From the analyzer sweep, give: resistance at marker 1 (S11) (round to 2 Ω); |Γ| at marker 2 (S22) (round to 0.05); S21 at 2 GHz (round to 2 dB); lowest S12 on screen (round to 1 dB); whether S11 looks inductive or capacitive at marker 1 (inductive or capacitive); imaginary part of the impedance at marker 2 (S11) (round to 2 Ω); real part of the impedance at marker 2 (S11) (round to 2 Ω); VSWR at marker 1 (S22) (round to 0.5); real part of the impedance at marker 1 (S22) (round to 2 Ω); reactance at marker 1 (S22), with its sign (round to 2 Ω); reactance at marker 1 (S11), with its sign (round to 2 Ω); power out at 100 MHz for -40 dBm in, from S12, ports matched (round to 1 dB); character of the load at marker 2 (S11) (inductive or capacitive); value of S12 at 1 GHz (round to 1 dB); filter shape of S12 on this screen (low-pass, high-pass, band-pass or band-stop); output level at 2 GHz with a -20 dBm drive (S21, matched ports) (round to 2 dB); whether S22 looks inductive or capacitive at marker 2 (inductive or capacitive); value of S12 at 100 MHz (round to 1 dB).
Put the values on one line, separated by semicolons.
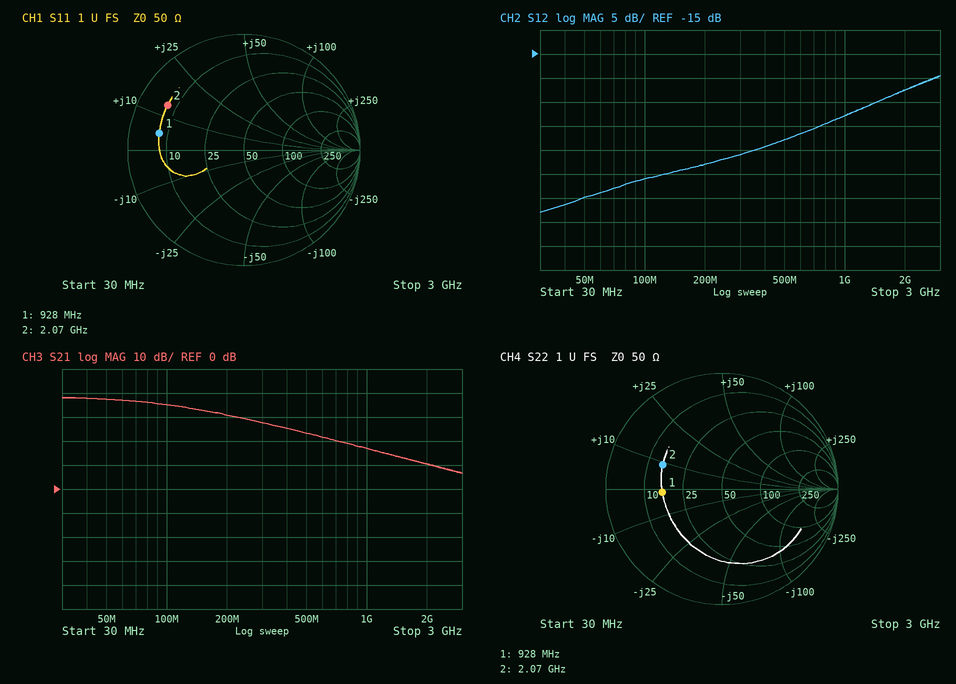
8 Ω; 0.55; 10 dB; -48 dB; inductive; +14 Ω; 8 Ω; 3.0; 16 Ω; -2 Ω; +4 Ω; -81 dBm; inductive; -28 dB; high-pass; -10 dBm; inductive; -41 dB
